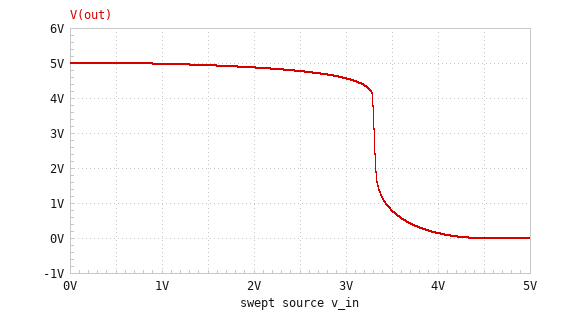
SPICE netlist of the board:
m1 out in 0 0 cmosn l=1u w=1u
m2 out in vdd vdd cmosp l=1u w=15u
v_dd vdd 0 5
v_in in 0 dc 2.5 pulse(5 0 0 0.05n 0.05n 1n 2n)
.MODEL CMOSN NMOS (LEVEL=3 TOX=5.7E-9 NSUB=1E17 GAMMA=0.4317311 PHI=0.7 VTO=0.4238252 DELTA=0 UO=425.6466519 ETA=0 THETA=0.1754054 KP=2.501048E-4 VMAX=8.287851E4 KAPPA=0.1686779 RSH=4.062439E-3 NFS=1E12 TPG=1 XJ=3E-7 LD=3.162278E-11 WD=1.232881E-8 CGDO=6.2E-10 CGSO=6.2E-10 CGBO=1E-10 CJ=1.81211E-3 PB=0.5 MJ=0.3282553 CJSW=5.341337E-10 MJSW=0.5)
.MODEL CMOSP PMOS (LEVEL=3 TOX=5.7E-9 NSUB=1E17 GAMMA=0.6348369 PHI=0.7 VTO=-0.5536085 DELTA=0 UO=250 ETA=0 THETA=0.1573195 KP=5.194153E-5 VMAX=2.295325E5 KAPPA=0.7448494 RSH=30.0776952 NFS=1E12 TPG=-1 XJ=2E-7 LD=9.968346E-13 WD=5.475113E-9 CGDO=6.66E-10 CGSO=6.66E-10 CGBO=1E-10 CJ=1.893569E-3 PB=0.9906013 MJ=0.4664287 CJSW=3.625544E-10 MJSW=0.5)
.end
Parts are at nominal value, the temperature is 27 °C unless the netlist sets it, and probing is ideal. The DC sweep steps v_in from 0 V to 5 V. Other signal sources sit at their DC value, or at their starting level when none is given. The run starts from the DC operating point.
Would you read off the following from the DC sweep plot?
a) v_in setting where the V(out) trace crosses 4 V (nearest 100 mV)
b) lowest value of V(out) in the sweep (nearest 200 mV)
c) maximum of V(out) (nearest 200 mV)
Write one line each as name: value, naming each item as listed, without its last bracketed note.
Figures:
v_in setting where the V(out) trace crosses 4 V: 3.3 V
lowest value of V(out) in the sweep: 0 V
maximum of V(out): 5.0 V
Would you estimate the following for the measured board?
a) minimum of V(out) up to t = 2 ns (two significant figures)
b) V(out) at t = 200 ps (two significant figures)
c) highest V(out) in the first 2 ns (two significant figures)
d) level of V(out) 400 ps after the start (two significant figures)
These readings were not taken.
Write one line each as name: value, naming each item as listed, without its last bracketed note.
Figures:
minimum of V(out) up to t = 2 ns: -660 mV
V(out) at t = 200 ps: 5.0 V
highest V(out) in the first 2 ns: 5.7 V
level of V(out) 400 ps after the start: 5.0 V
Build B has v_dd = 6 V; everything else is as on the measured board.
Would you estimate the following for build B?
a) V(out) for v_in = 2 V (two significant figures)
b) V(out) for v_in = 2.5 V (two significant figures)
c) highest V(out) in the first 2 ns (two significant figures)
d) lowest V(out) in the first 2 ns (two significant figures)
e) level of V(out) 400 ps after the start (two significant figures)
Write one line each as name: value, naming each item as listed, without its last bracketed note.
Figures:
V(out) for v_in = 2 V: 5.9 V
V(out) for v_in = 2.5 V: 5.8 V
highest V(out) in the first 2 ns: 6.7 V
lowest V(out) in the first 2 ns: -640 mV
level of V(out) 400 ps after the start: 6.0 V
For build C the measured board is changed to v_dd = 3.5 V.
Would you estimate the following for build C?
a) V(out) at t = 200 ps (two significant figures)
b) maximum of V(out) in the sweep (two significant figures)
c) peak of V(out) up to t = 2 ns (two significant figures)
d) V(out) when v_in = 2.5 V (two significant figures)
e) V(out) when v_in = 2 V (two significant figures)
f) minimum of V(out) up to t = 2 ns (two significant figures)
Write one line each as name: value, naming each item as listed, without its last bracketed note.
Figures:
V(out) at t = 200 ps: 3.4 V
maximum of V(out) in the sweep: 3.5 V
peak of V(out) up to t = 2 ns: 4.2 V
V(out) when v_in = 2.5 V: 220 mV
V(out) when v_in = 2 V: 3.2 V
minimum of V(out) up to t = 2 ns: -660 mV
